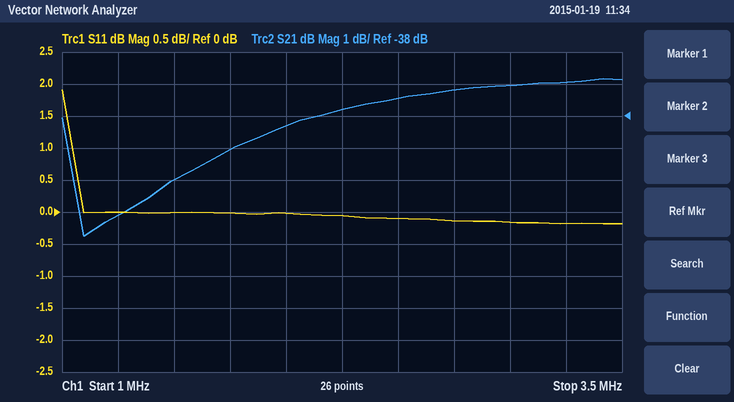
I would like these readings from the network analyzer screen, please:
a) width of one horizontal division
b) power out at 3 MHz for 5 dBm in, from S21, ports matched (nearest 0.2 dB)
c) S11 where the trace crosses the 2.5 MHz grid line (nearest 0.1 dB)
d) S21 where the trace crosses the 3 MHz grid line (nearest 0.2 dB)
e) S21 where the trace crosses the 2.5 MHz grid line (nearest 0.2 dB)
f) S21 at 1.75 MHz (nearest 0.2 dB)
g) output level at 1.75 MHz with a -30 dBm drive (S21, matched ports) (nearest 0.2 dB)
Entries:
250 kHz
-32.0 dBm
-0.1 dB
-37.0 dB
-37.4 dB
-39.0 dB
-69.0 dBm
